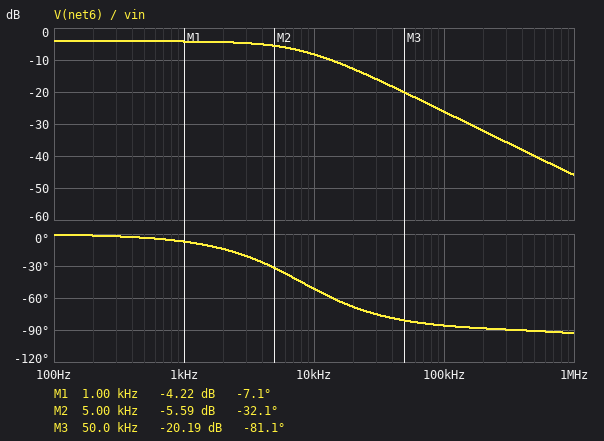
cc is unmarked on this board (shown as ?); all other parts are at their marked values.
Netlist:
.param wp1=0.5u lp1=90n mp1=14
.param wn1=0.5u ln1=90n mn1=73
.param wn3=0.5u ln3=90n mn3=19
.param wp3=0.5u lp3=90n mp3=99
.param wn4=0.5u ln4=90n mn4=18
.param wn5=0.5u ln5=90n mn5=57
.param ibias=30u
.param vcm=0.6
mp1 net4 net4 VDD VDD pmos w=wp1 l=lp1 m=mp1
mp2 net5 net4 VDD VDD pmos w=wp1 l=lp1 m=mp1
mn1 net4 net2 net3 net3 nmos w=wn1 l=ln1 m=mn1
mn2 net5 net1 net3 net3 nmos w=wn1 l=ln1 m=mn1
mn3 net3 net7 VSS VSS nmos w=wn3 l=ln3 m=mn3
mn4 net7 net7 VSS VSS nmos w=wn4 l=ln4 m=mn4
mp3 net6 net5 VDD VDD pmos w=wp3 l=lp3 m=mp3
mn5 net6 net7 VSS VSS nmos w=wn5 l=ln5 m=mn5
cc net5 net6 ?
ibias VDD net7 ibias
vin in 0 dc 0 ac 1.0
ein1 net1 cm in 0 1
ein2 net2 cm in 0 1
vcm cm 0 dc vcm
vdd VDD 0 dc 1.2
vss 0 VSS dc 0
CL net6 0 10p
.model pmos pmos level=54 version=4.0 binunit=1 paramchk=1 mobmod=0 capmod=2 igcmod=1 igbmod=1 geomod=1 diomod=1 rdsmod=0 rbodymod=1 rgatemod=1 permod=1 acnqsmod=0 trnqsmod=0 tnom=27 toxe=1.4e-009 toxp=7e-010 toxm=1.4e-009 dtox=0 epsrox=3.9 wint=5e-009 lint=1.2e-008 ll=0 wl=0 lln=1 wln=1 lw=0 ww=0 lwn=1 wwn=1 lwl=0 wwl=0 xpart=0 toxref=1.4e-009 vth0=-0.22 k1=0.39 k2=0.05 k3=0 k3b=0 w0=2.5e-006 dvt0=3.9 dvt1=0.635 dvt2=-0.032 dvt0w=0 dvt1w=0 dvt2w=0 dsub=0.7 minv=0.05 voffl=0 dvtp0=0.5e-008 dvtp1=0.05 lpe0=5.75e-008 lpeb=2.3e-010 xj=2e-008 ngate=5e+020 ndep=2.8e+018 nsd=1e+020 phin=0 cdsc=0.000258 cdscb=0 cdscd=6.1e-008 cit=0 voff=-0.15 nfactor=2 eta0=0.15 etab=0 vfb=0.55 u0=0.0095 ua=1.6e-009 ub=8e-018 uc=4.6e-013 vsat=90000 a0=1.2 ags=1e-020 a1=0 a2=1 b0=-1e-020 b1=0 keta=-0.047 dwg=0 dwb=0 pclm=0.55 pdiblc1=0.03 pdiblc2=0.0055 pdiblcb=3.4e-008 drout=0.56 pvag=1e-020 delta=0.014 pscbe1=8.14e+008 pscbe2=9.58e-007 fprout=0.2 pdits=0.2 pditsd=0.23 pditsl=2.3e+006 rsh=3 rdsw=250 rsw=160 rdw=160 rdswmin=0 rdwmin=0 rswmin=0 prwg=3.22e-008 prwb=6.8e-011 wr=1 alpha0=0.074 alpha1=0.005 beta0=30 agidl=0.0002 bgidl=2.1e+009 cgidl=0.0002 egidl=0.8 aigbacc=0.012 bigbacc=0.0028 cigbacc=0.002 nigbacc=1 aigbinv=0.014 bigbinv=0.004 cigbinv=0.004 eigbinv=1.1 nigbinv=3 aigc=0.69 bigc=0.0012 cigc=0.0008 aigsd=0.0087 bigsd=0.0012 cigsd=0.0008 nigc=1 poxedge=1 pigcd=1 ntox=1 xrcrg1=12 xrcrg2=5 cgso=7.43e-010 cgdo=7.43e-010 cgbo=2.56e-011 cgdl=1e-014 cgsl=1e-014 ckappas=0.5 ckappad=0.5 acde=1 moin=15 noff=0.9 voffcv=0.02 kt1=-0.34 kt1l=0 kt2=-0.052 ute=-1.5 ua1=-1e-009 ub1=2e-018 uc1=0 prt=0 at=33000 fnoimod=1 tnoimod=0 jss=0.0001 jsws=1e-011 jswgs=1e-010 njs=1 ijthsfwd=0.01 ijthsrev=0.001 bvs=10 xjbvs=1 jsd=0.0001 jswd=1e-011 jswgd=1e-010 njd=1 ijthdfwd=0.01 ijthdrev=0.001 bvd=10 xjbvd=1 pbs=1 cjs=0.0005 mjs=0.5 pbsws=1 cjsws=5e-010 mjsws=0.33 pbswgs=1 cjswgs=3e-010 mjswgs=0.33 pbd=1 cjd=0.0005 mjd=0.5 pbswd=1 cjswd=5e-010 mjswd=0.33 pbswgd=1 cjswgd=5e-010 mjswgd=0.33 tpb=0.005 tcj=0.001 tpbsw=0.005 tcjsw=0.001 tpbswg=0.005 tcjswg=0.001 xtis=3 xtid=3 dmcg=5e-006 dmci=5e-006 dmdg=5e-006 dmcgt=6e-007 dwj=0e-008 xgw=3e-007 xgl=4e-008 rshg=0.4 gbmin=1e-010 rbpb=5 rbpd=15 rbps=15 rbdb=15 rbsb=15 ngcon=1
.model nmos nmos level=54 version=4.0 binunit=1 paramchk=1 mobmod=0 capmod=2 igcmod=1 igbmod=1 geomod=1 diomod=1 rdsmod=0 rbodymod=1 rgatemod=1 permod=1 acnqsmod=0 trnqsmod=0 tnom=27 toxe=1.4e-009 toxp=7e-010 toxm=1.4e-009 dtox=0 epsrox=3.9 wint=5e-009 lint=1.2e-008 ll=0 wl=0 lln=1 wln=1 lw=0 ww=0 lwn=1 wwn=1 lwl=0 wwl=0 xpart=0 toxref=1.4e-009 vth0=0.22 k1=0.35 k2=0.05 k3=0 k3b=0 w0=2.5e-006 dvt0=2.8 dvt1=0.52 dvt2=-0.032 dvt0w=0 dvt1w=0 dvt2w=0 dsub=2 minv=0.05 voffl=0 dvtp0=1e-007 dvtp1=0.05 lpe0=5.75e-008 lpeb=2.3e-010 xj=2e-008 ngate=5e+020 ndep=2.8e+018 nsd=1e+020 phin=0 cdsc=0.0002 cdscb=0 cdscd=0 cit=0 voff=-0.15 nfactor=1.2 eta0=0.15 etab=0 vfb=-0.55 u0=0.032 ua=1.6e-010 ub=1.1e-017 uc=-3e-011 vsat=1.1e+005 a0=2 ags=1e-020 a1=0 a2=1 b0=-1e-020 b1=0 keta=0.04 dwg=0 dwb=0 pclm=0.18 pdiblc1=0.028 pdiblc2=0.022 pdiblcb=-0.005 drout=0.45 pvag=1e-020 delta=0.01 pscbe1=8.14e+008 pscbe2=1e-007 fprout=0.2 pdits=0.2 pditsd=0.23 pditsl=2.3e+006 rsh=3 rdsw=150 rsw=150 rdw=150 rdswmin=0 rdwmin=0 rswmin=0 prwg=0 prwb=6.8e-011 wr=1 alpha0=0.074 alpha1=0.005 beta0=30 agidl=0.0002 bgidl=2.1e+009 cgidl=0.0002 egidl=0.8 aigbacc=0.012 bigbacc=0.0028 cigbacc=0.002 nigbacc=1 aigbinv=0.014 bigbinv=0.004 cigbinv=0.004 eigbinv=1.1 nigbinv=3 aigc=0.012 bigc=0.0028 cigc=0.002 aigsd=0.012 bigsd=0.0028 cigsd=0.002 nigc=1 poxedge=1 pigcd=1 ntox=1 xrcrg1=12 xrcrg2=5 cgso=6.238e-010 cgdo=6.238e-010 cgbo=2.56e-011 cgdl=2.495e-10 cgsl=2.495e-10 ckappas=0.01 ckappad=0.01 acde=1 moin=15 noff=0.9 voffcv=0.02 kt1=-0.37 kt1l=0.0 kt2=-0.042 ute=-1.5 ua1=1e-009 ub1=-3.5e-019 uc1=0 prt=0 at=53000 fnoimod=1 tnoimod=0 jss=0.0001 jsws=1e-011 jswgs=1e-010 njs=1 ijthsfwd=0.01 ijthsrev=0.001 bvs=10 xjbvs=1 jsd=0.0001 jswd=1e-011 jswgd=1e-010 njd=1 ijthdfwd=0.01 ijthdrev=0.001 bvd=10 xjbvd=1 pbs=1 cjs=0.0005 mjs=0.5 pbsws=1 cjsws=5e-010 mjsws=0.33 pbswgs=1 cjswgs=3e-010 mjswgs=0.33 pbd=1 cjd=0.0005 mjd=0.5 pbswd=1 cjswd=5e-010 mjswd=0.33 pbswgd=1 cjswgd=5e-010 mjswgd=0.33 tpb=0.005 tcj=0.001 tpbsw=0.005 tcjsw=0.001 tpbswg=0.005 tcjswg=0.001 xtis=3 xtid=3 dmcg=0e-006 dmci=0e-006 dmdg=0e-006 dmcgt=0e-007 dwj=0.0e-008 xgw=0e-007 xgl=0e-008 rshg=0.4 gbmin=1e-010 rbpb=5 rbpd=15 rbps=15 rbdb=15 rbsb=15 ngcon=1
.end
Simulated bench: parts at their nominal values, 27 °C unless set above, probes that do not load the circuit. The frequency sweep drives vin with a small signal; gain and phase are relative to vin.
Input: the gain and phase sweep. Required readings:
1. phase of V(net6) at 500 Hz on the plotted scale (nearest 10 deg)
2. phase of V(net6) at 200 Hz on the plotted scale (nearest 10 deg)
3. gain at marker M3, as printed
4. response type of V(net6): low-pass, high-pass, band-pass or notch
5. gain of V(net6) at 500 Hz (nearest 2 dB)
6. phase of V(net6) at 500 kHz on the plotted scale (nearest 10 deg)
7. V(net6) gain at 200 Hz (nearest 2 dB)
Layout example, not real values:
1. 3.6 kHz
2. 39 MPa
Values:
1. 0 deg
2. 0 deg
3. -20.19 dB
4. low-pass
5. -4 dB
6. -90 deg
7. -4 dB
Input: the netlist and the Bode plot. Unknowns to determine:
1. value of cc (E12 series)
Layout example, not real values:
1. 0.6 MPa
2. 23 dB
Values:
1. 18 pF
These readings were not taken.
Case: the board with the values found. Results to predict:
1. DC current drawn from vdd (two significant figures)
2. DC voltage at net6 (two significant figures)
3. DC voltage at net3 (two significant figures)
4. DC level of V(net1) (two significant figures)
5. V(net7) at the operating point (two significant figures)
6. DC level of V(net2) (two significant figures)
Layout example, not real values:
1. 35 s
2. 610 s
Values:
1. 180 µA
2. 690 mV
3. 350 mV
4. 600 mV
5. 350 mV
6. 600 mV
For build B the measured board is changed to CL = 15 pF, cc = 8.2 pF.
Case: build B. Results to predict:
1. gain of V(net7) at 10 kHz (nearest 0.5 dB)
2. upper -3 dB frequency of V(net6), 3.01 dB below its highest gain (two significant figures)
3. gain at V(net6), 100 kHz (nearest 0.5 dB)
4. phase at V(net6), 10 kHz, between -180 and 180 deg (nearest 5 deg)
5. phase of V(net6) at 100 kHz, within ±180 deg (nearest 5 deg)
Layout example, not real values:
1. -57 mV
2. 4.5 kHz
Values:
1. -60.0 dB
2. 17 kHz
3. -19.5 dB
4. -30 deg
5. -80 deg
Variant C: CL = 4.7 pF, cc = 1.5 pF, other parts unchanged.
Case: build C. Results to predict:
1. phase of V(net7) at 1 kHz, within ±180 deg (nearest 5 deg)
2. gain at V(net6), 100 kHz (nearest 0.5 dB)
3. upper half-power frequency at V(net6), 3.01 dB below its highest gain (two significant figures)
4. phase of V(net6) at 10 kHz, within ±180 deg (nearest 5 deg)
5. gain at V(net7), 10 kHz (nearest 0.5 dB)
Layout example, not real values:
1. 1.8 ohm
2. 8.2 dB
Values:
1. 0 deg
2. -7.5 dB
3. 91 kHz
4. -5 deg
5. -59.0 dB
